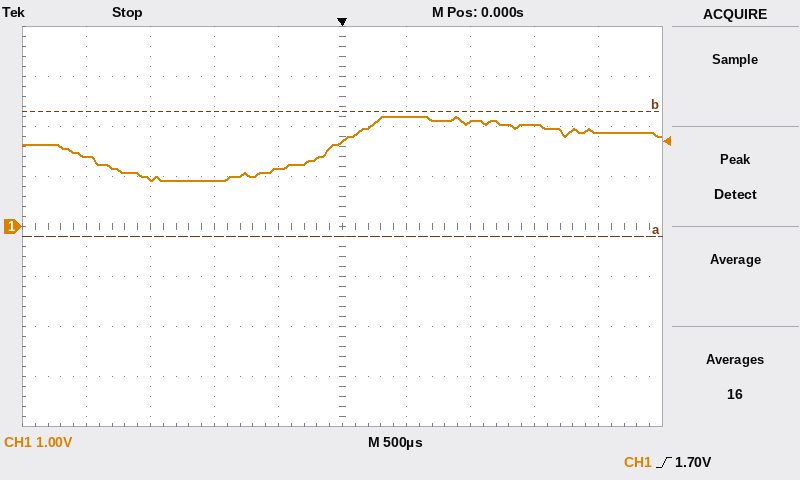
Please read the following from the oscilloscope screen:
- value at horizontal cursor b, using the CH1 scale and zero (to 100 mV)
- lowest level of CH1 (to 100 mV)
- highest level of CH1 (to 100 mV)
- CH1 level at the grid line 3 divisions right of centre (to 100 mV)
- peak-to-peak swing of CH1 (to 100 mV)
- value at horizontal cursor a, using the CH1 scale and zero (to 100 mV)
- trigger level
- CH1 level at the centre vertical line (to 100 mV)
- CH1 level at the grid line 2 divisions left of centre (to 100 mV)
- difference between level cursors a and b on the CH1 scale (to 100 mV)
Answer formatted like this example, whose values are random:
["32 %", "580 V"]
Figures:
["2.3 V", "900 mV", "2.2 V", "2.0 V", "1.3 V", "-200 mV", "1.70 V", "1.7 V", "900 mV", "2.5 V"]
